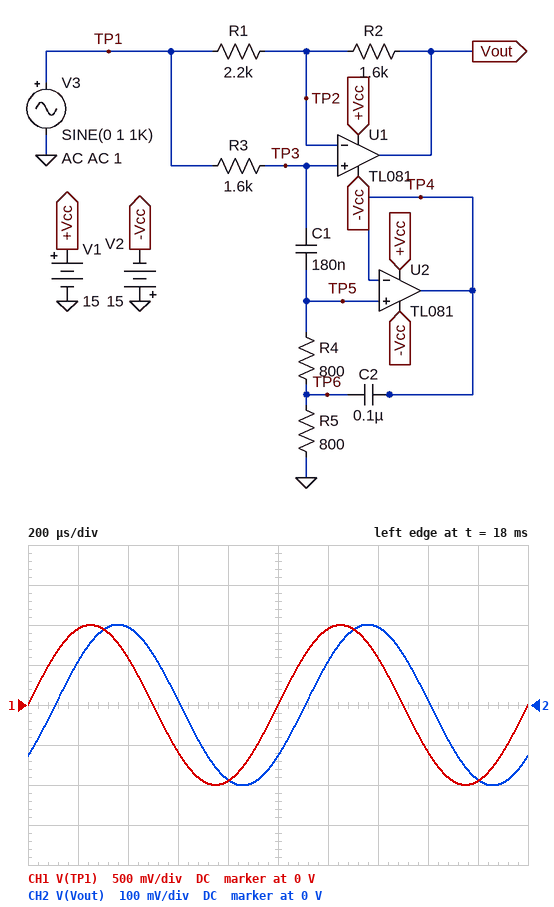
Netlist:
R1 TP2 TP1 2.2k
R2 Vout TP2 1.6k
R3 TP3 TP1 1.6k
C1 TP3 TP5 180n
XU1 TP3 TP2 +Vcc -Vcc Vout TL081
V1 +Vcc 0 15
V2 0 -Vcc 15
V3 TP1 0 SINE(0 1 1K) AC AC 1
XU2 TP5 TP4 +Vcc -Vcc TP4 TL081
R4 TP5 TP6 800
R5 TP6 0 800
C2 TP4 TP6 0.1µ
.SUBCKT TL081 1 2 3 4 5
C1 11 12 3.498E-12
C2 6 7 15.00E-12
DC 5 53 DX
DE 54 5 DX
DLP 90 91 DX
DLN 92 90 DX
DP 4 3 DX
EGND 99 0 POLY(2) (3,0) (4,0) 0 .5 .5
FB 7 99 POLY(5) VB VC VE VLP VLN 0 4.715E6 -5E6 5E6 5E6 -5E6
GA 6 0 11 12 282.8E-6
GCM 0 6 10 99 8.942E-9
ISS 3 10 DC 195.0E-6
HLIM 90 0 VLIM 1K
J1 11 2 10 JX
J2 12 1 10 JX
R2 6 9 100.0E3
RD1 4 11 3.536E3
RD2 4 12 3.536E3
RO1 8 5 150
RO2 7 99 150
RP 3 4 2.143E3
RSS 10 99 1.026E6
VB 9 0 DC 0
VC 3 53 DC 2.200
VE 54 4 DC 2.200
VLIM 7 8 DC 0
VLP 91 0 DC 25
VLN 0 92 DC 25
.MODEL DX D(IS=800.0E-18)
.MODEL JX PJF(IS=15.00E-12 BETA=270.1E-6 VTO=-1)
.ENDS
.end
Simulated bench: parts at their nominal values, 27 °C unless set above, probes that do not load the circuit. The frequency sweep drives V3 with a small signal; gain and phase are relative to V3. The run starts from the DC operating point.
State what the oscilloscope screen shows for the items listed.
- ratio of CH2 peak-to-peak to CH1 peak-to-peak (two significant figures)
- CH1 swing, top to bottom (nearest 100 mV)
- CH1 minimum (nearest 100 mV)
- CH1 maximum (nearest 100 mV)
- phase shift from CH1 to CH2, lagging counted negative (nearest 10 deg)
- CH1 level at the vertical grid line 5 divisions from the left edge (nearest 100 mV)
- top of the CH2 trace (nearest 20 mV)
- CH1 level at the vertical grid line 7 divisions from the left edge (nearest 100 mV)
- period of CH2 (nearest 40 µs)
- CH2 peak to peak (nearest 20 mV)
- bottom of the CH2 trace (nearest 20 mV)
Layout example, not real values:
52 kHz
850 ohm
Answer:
0.20
2.0 V
-1.0 V
1.0 V
-40 deg
0 V
200 mV
600 mV
1.00 ms
400 mV
-200 mV
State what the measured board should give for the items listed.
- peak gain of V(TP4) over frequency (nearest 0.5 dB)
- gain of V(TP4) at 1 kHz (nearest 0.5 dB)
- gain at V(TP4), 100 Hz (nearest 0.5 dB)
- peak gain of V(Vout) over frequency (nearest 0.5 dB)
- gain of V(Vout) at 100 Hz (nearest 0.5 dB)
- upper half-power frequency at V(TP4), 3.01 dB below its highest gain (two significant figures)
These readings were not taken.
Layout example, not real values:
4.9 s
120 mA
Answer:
0 dB
-6.0 dB
-15.5 dB
0 dB
-0.5 dB
1.1 MHz
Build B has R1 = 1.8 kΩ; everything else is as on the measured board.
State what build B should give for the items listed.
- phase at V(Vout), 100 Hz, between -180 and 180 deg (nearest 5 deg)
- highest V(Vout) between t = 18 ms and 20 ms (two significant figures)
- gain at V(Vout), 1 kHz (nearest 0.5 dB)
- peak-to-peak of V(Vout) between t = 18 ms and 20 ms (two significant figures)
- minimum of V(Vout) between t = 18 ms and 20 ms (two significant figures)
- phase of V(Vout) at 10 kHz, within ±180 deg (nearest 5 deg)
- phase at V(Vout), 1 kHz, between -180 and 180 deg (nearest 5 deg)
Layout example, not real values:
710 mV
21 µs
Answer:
-20 deg
160 mV
-16.0 dB
320 mV
-160 mV
35 deg
-60 deg
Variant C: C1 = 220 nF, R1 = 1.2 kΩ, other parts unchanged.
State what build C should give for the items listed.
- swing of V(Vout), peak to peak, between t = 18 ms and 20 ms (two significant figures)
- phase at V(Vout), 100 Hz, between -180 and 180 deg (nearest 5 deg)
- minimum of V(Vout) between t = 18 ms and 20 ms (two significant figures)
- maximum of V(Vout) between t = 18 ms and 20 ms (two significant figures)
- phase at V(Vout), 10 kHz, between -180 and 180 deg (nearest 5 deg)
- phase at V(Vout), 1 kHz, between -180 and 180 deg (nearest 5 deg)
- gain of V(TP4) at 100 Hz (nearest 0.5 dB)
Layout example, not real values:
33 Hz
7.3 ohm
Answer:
390 mV
-30 deg
-190 mV
190 mV
45 deg
-145 deg
-14.0 dB
